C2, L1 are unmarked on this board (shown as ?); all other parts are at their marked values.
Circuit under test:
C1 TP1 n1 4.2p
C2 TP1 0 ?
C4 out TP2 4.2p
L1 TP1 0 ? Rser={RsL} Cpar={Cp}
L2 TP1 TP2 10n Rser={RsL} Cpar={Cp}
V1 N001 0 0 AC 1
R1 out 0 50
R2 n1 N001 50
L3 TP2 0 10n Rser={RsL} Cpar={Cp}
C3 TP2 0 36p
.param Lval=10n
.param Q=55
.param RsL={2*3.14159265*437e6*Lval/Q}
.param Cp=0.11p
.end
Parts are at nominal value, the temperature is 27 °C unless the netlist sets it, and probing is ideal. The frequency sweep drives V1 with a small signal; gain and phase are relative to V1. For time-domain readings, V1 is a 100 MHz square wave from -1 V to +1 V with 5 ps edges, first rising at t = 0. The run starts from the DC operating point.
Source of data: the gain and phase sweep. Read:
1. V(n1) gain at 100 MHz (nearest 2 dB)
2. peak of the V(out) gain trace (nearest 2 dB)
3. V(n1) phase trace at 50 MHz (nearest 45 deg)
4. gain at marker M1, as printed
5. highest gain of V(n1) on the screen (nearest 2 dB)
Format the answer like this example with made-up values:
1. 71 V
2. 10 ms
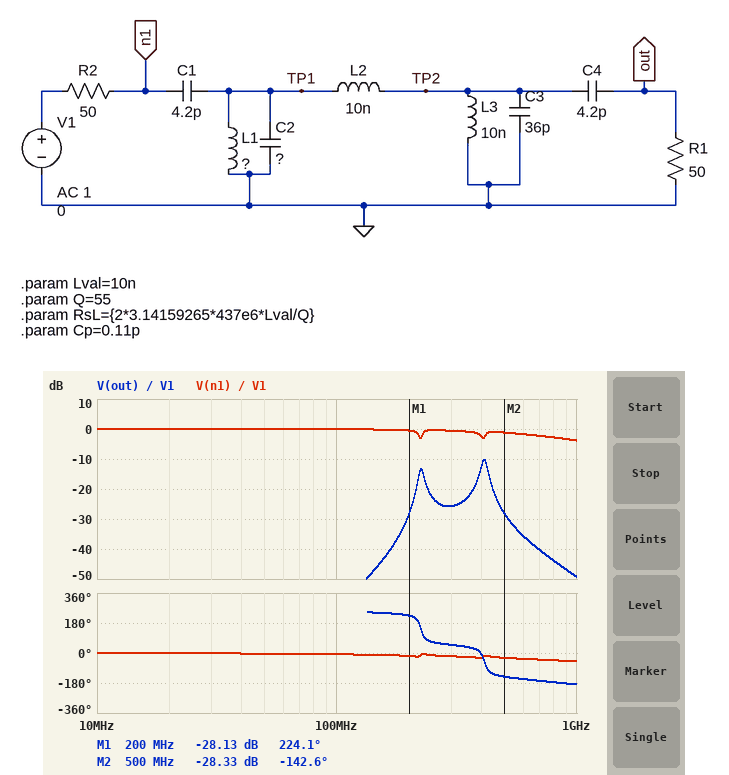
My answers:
1. 0 dB
2. -10 dB
3. 0 deg
4. -28.13 dB
5. 0 dB
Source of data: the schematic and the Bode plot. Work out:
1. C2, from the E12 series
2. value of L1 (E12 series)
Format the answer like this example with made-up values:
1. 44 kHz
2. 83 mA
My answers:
1. 47 pF
2. 12 nH
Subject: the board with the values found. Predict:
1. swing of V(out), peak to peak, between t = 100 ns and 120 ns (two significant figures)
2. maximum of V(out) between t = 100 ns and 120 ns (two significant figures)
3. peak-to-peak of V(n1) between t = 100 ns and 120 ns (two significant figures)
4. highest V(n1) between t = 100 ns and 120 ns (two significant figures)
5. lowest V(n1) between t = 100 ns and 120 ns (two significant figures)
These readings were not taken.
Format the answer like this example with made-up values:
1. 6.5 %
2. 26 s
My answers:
1. 61 mV
2. 31 mV
3. 2.0 V
4. 1.0 V
5. -1.0 V
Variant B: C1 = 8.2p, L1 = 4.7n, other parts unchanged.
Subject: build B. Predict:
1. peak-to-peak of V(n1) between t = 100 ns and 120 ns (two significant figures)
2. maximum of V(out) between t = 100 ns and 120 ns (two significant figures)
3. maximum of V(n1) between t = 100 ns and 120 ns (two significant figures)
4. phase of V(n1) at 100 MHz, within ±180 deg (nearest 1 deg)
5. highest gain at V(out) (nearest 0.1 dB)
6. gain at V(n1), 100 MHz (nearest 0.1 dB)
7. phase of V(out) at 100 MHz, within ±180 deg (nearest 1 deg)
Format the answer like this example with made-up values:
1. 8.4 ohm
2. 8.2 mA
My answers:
1. 2.1 V
2. 120 mV
3. 1.1 V
4. -15 deg
5. -9.8 dB
6. -0.3 dB
7. -122 deg
